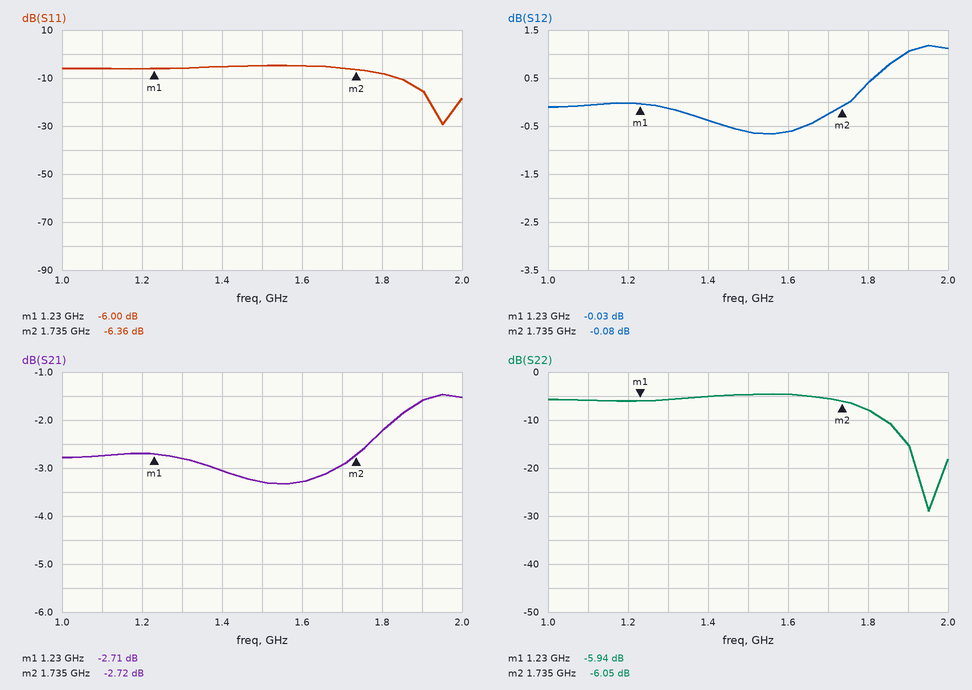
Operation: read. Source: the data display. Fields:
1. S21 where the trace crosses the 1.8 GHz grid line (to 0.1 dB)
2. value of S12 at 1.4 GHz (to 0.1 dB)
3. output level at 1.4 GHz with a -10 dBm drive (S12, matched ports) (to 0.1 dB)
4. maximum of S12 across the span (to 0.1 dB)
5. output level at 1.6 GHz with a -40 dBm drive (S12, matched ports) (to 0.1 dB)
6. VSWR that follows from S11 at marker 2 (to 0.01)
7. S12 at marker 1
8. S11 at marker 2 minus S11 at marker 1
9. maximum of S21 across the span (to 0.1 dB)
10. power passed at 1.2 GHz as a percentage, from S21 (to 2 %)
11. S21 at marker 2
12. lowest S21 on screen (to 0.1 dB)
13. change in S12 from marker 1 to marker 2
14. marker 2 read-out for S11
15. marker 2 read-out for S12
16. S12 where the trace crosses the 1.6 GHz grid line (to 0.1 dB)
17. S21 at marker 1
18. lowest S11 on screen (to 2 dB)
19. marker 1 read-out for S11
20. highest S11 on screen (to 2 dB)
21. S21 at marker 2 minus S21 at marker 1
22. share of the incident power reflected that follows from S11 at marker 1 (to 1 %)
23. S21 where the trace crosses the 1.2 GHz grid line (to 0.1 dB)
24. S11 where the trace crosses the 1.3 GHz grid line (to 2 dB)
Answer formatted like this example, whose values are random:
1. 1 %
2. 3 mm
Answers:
1. -2.2 dB
2. -0.4 dB
3. -10.4 dBm
4. 1.2 dB
5. -40.6 dBm
6. 2.85
7. -0.03 dB
8. -0.36 dB
9. -1.5 dB
10. 54 %
11. -2.72 dB
12. -3.3 dB
13. -0.05 dB
14. -6.36 dB
15. -0.08 dB
16. -0.6 dB
17. -2.71 dB
18. -30 dB
19. -6.00 dB
20. -4 dB
21. -0.01 dB
22. 25 %
23. -2.7 dB
24. -6 dB
